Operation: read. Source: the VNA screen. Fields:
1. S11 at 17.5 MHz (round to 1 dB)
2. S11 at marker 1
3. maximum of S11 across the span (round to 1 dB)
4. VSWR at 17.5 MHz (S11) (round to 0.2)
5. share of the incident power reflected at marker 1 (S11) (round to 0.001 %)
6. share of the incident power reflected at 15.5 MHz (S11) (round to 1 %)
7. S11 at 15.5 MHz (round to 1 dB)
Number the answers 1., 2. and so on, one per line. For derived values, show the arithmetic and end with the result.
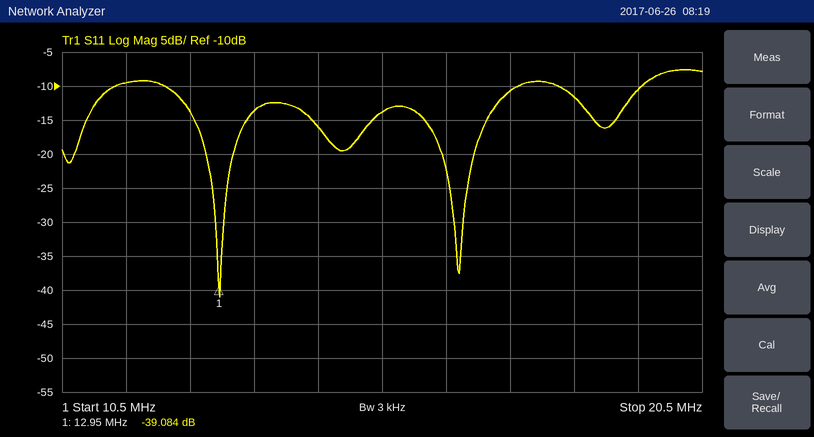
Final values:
1. -11 dB
2. -39.084 dB
3. -8 dB
4. |Γ| = 10^(-11/20) = 0.2818; VSWR = (1 + 0.2818)/(1 − 0.2818) ≈ 1.8
5. 10^(-39.084/10) ≈ 0.012 %
6. 10^(-14/10) ≈ 4 %
7. -14 dB
